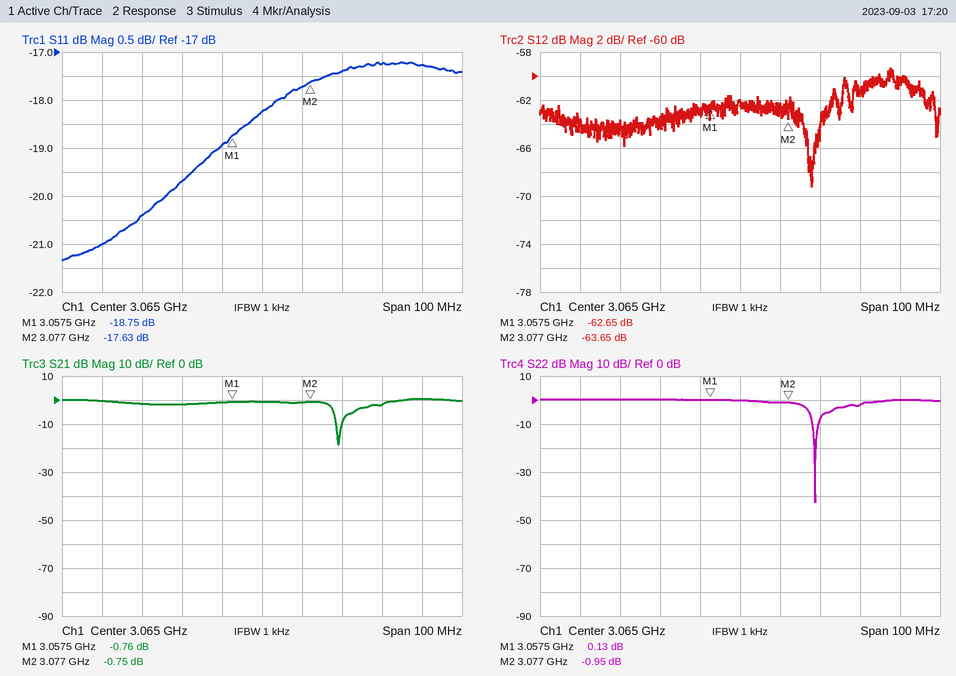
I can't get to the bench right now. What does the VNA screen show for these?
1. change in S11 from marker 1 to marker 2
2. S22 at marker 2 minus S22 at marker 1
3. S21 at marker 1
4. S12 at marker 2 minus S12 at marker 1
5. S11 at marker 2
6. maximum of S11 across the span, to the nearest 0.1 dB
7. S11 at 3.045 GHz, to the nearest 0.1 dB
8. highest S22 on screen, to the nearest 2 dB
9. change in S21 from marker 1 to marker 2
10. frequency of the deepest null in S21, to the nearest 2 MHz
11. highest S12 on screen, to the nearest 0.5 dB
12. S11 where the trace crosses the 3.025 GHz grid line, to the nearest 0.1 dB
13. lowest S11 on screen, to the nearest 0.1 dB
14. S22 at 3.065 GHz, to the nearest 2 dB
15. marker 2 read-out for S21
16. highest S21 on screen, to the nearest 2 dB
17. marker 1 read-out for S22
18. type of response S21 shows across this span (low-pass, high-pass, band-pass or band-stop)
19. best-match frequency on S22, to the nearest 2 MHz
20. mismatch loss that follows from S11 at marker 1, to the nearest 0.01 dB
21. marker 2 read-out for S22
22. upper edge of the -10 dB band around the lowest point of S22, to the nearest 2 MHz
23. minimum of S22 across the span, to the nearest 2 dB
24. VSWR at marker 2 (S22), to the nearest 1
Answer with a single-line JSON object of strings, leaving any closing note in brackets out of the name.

{"change in S11 from marker 1 to marker 2": "1.12 dB", "S22 at marker 2 minus S22 at marker 1": "-1.08 dB", "S21 at marker 1": "-0.76 dB", "S12 at marker 2 minus S12 at marker 1": "-1.00 dB", "S11 at marker 2": "-17.63 dB", "maximum of S11 across the span, to the nearest 0.1 dB": "-17.2 dB", "S11 at 3.045 GHz, to the nearest 0.1 dB": "-19.7 dB", "highest S22 on screen, to the nearest 2 dB": "0 dB", "change in S21 from marker 1 to marker 2": "0.01 dB", "frequency of the deepest null in S21, to the nearest 2 MHz": "3.084 GHz", "highest S12 on screen, to the nearest 0.5 dB": "-59.5 dB", "S11 where the trace crosses the 3.025 GHz grid line, to the nearest 0.1 dB": "-21.0 dB", "lowest S11 on screen, to the nearest 0.1 dB": "-21.3 dB", "S22 at 3.065 GHz, to the nearest 2 dB": "0 dB", "marker 2 read-out for S21": "-0.75 dB", "highest S21 on screen, to the nearest 2 dB": "0 dB", "marker 1 read-out for S22": "0.13 dB", "type of response S21 shows across this span": "band-stop", "best-match frequency on S22, to the nearest 2 MHz": "3.084 GHz", "mismatch loss that follows from S11 at marker 1, to the nearest 0.01 dB": "0.06 dB", "marker 2 read-out for S22": "-0.95 dB", "upper edge of the -10 dB band around the lowest point of S22, to the nearest 2 MHz": "3.084 GHz", "minimum of S22 across the span, to the nearest 2 dB": "-42 dB", "VSWR at marker 2 (S22), to the nearest 1": "18"}
